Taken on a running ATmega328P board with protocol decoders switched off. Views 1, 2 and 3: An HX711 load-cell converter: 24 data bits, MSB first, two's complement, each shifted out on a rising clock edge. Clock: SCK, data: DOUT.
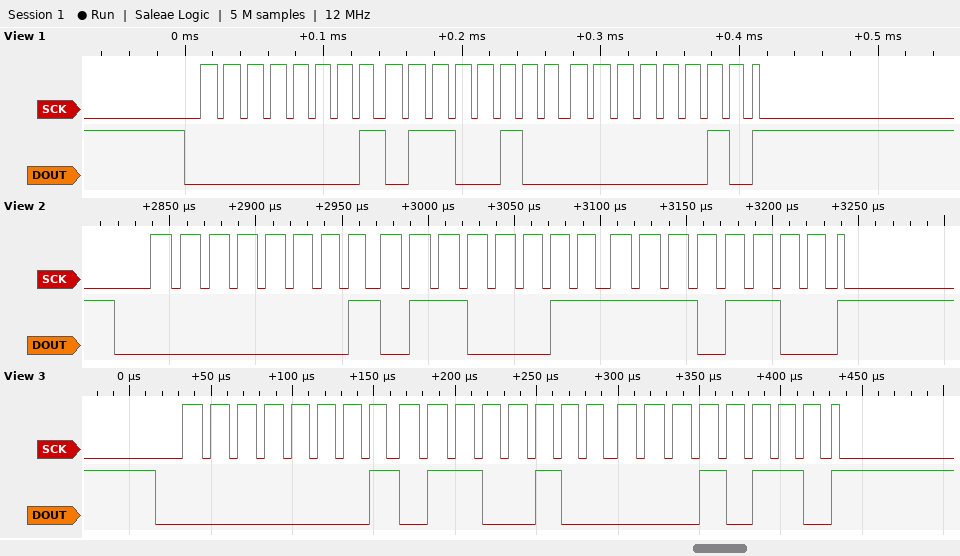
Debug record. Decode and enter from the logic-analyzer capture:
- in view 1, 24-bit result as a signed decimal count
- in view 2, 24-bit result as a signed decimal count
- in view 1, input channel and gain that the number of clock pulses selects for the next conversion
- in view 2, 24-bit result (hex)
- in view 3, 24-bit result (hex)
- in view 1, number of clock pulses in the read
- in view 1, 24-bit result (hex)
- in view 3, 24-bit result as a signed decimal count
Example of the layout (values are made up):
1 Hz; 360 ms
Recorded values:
91138; 91116; channel A, gain 128; 0x0163EC; 0x016416; 25; 0x016402; 91158
